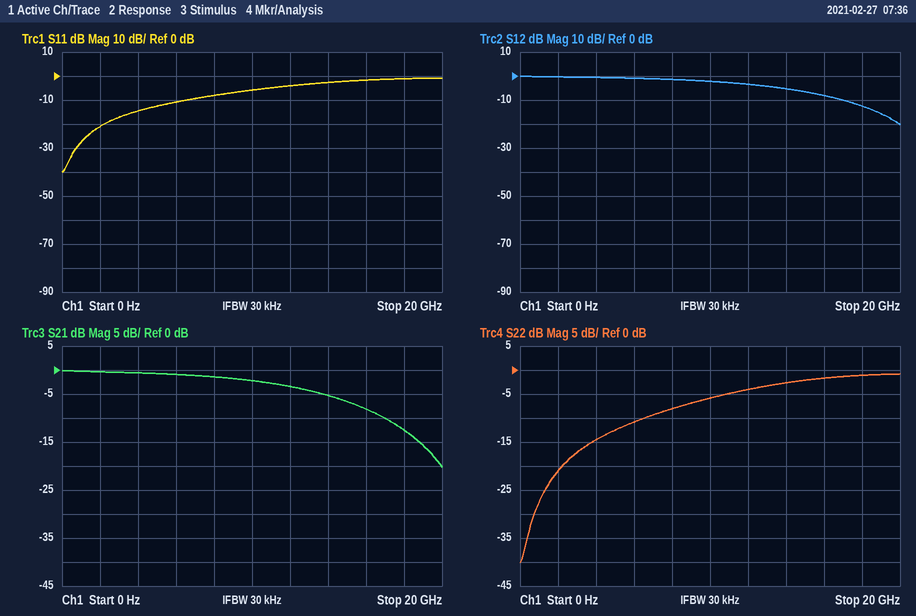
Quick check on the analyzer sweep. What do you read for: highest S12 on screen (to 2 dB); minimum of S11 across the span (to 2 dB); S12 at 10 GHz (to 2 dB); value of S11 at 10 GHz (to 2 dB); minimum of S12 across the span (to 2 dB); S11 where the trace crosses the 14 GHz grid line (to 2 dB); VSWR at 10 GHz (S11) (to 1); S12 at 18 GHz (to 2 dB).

0 dB
-40 dB
-2 dB
-6 dB
-20 dB
-2 dB
3
-12 dB
